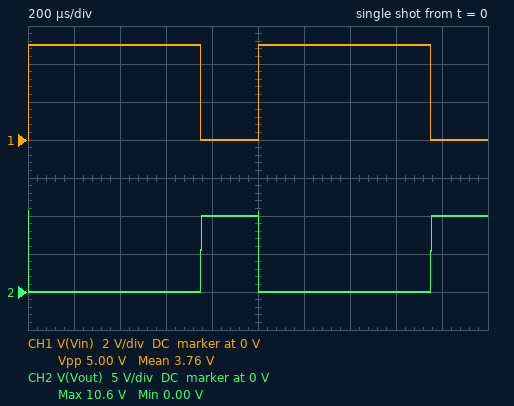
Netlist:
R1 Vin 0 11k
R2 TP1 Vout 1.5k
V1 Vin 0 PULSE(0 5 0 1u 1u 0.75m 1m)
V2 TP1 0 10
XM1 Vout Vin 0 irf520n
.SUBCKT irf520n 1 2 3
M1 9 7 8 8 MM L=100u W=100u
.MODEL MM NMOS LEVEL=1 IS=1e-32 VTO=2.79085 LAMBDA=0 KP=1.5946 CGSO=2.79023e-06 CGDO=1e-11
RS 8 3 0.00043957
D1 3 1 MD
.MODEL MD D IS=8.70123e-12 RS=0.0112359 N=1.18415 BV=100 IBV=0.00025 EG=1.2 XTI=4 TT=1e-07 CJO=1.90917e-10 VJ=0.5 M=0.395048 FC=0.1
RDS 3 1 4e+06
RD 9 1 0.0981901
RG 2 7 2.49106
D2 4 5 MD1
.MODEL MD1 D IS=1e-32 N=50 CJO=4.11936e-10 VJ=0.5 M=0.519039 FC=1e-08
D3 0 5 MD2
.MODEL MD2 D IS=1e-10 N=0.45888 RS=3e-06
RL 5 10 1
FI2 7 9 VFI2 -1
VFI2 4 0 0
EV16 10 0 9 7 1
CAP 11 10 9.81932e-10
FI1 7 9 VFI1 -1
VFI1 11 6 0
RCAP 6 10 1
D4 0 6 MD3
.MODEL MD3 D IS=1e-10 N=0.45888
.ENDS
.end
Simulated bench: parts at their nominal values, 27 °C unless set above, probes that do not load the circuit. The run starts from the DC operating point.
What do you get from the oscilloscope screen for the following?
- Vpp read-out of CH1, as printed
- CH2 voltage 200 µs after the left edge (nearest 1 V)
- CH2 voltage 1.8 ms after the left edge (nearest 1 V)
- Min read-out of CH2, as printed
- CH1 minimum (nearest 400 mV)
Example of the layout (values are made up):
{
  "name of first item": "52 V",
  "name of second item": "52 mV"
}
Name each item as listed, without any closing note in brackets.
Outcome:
{
  "Vpp read-out of CH1, as printed": "5.00 V",
  "CH2 voltage 200 µs after the left edge": "0 V",
  "CH2 voltage 1.8 ms after the left edge": "10 V",
  "Min read-out of CH2, as printed": "0.00 V",
  "CH1 minimum": "0 V"
}
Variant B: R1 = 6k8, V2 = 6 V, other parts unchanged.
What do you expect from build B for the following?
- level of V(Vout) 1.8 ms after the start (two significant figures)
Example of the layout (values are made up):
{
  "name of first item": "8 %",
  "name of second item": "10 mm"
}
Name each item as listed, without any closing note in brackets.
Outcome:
{
  "level of V(Vout) 1.8 ms after the start": "6.0 V"
}
